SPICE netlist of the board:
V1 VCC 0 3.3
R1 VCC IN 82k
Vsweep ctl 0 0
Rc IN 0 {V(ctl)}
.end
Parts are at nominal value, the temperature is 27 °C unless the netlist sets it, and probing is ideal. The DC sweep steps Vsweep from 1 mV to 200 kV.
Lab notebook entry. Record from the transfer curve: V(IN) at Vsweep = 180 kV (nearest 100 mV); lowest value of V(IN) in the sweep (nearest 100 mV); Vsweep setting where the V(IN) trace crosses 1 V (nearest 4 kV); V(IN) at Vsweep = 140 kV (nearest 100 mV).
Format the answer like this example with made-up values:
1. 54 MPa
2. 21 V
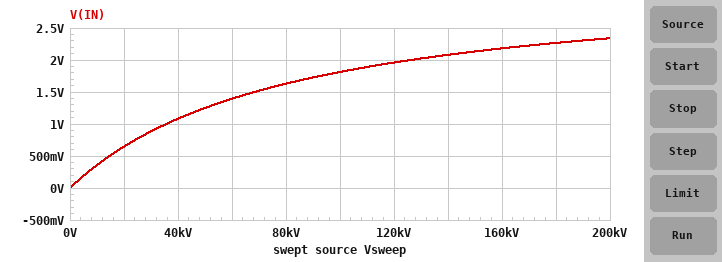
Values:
1. 2.3 V
2. 0 V
3. 36 kV
4. 2.1 V
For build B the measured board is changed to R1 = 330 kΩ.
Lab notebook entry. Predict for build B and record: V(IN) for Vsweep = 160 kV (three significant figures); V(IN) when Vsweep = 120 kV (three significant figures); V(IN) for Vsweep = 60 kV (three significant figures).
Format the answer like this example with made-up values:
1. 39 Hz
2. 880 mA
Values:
1. 1.08 V
2. 880 mV
3. 508 mV
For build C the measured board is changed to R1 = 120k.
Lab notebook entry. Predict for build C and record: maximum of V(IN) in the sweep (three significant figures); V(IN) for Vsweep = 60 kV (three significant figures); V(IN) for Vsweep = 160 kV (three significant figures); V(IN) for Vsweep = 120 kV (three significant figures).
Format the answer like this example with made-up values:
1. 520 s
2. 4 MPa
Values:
1. 2.06 V
2. 1.10 V
3. 1.89 V
4. 1.65 V
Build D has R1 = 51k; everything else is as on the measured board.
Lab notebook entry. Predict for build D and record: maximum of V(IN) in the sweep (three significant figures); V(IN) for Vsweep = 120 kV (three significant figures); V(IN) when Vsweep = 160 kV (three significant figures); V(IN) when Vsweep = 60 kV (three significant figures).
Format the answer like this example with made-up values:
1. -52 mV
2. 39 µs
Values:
1. 2.63 V
2. 2.32 V
3. 2.50 V
4. 1.78 V
